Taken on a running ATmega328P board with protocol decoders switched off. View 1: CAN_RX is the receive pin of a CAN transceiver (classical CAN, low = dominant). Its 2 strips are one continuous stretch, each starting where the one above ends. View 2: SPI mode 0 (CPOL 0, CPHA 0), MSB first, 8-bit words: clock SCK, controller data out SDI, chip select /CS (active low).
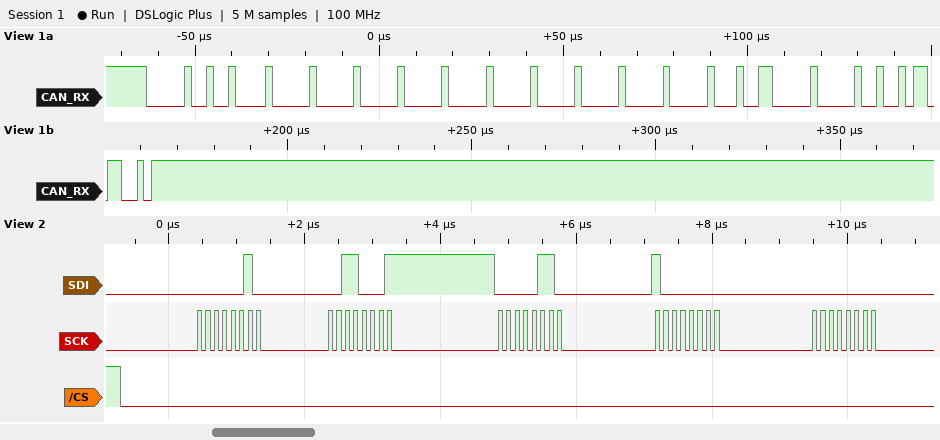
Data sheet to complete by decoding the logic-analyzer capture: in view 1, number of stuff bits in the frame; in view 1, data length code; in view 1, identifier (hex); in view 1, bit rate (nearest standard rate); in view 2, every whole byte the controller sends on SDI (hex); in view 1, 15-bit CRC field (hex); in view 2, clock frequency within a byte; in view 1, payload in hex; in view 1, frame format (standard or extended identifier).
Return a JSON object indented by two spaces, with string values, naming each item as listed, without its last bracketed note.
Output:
{
  "in view 1, number of stuff bits in the frame": "13",
  "in view 1, data length code": "8",
  "in view 1, identifier": "0x012",
  "in view 1, bit rate": "500 kbit/s",
  "in view 2, every whole byte the controller sends on SDI": "02 31 06 80 00",
  "in view 1, 15-bit CRC field": "0x096C",
  "in view 2, clock frequency within a byte": "8 MHz",
  "in view 1, payload in hex": "00 00 00 00 00 00 26 00",
  "in view 1, frame format": "standard"
}
